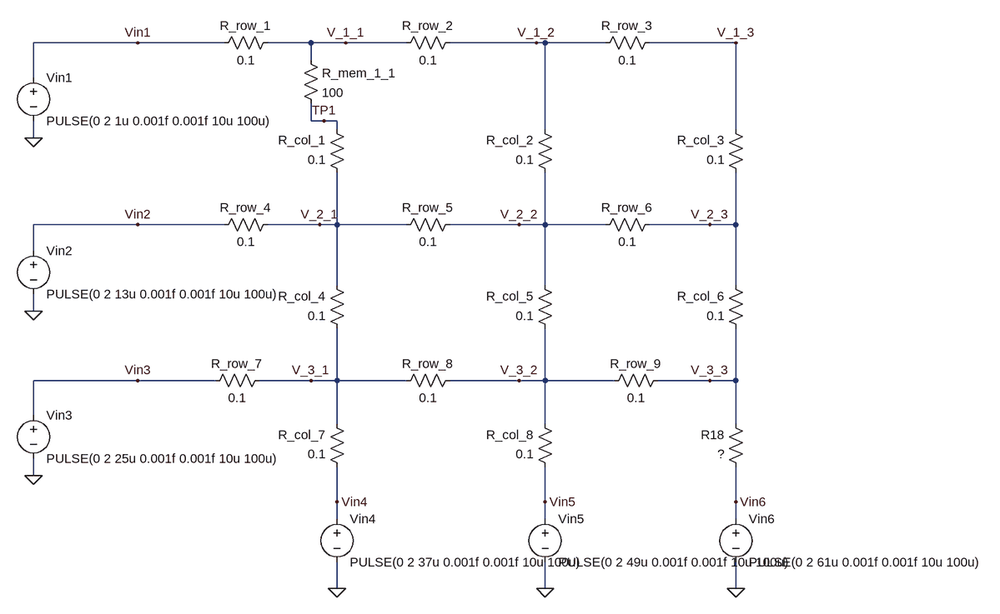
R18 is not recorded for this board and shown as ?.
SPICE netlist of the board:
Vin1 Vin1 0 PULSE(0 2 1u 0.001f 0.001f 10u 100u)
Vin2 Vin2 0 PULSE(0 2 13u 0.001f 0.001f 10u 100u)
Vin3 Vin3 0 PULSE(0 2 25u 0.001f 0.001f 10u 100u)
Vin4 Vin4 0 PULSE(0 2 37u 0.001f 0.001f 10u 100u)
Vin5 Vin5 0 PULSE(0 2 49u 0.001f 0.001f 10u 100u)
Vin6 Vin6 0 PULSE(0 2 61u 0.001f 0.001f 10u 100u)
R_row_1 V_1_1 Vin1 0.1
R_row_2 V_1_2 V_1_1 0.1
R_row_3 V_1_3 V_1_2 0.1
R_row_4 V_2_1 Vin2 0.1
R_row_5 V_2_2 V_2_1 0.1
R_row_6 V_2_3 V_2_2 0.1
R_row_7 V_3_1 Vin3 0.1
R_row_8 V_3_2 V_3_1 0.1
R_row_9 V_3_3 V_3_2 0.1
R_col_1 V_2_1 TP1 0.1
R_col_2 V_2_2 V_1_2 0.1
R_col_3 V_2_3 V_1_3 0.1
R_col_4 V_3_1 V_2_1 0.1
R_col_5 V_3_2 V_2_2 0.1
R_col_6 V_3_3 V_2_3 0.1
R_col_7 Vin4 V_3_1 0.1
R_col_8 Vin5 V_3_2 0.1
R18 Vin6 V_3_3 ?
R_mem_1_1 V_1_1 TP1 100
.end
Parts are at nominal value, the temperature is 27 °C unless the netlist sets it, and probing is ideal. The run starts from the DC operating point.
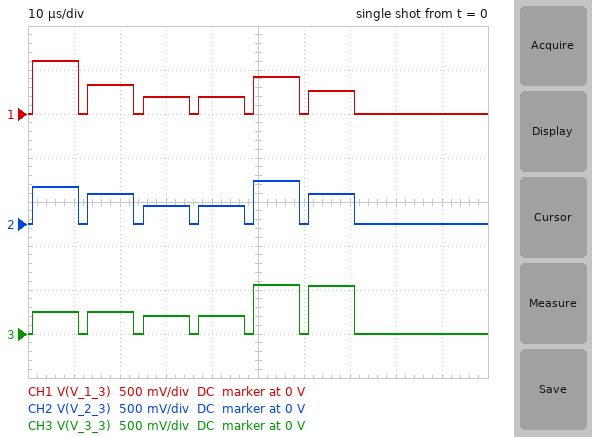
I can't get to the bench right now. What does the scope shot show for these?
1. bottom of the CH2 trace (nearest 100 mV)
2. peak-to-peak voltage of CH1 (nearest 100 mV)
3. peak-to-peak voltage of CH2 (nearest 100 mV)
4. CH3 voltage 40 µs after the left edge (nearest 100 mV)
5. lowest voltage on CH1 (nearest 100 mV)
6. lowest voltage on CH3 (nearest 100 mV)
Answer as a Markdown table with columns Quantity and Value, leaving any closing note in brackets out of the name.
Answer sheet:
| Quantity | Value |
|---|---|
| bottom of the CH2 trace | 0 V |
| peak-to-peak voltage of CH1 | 600 mV |
| peak-to-peak voltage of CH2 | 500 mV |
| CH3 voltage 40 µs after the left edge | 200 mV |
| lowest voltage on CH1 | 0 V |
| lowest voltage on CH3 | 0 V |
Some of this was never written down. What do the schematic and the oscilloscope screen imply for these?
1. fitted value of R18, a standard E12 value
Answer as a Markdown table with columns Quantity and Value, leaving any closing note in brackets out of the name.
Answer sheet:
| Quantity | Value |
|---|---|
| fitted value of R18, a standard E12 value | 0.27 Ω |
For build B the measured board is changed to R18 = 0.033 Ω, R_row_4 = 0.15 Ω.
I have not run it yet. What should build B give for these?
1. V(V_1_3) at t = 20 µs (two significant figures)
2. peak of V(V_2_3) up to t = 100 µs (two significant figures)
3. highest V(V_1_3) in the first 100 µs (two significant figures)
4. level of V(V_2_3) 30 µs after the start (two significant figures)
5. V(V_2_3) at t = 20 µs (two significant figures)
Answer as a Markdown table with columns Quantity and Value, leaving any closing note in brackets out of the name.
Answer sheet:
| Quantity | Value |
|---|---|
| V(V_1_3) at t = 20 µs | 200 mV |
| peak of V(V_2_3) up to t = 100 µs | 950 mV |
| highest V(V_1_3) in the first 100 µs | 740 mV |
| level of V(V_2_3) 30 µs after the start | 140 mV |
| V(V_2_3) at t = 20 µs | 190 mV |
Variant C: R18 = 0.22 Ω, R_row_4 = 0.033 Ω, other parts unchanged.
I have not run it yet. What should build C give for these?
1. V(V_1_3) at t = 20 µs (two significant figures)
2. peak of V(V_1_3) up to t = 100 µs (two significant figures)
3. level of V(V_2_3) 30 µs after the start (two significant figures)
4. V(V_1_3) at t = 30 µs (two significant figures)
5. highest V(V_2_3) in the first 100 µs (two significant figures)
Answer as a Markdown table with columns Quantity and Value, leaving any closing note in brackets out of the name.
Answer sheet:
| Quantity | Value |
|---|---|
| V(V_1_3) at t = 20 µs | 510 mV |
| peak of V(V_1_3) up to t = 100 µs | 570 mV |
| level of V(V_2_3) 30 µs after the start | 150 mV |
| V(V_1_3) at t = 30 µs | 130 mV |
| highest V(V_2_3) in the first 100 µs | 530 mV |
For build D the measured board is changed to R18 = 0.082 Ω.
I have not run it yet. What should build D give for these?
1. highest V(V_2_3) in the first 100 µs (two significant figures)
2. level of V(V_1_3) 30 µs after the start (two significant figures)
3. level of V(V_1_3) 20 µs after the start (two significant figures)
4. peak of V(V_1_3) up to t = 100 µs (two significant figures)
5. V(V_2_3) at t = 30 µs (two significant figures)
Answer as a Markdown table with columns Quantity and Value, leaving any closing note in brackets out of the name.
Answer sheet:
| Quantity | Value |
|---|---|
| highest V(V_2_3) in the first 100 µs | 680 mV |
| level of V(V_1_3) 30 µs after the start | 150 mV |
| level of V(V_1_3) 20 µs after the start | 280 mV |
| peak of V(V_1_3) up to t = 100 µs | 560 mV |
| V(V_2_3) at t = 30 µs | 160 mV |
